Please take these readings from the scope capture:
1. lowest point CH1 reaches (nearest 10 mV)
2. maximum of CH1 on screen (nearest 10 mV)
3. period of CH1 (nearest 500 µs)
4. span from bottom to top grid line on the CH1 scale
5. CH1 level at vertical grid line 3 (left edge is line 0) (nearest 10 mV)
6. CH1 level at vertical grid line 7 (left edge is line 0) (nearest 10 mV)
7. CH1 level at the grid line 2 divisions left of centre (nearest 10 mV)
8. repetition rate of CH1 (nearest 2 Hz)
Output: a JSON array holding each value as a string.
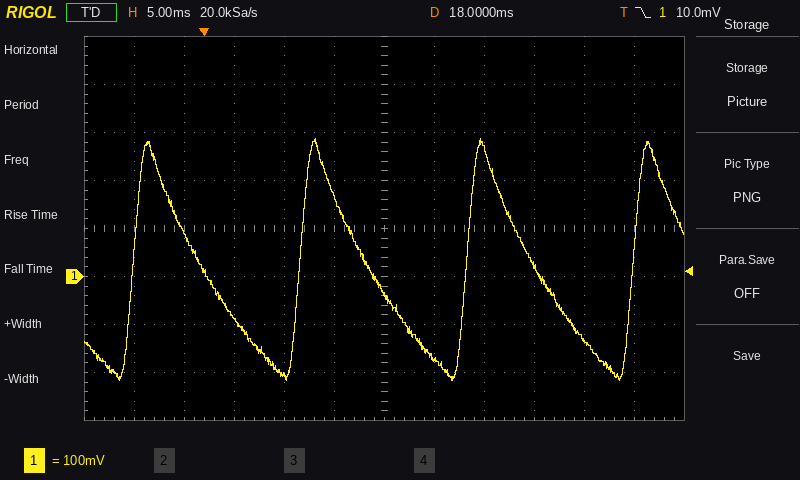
["-220 mV", "290 mV", "16.5 ms", "800 mV", "-90 mV", "-170 mV", "-210 mV", "60 Hz"]
